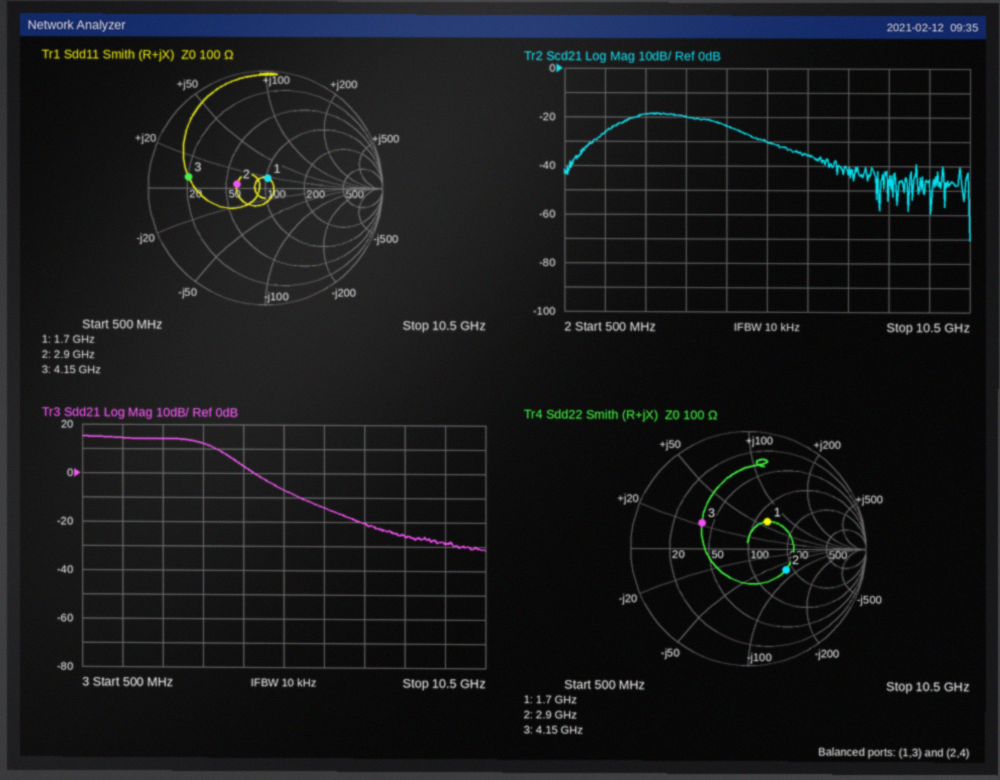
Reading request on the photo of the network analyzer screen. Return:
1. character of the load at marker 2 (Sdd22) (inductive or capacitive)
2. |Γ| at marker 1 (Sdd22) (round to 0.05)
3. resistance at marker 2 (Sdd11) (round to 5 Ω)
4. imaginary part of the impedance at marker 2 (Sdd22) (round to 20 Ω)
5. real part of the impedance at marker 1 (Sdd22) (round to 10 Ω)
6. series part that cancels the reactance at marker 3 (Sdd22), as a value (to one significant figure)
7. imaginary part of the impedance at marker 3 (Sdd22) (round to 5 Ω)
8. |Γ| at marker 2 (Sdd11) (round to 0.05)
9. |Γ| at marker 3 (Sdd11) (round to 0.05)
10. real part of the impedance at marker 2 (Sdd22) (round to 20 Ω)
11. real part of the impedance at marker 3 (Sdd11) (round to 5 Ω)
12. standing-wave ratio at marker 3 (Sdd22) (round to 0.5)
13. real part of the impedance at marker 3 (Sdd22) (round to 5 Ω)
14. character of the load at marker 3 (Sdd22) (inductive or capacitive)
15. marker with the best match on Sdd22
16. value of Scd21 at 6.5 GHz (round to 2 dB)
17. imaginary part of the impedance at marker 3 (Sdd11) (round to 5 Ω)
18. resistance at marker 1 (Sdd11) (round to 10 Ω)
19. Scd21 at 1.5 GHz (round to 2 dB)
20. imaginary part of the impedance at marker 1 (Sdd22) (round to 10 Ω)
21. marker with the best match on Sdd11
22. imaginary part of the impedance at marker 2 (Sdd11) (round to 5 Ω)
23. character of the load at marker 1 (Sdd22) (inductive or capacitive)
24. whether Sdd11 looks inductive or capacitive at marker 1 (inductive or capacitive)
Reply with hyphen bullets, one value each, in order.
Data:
- capacitive
- 0.30
- 60 Ω
- -80 Ω
- 120 Ω
- 2 pF
- +20 Ω
- 0.25
- 0.65
- 180 Ω
- 20 Ω
- 2.5
- 40 Ω
- inductive
- marker 1
- -36 dB
- +5 Ω
- 100 Ω
- -26 dB
- +60 Ω
- marker 1
- +5 Ω
- inductive
- inductive
